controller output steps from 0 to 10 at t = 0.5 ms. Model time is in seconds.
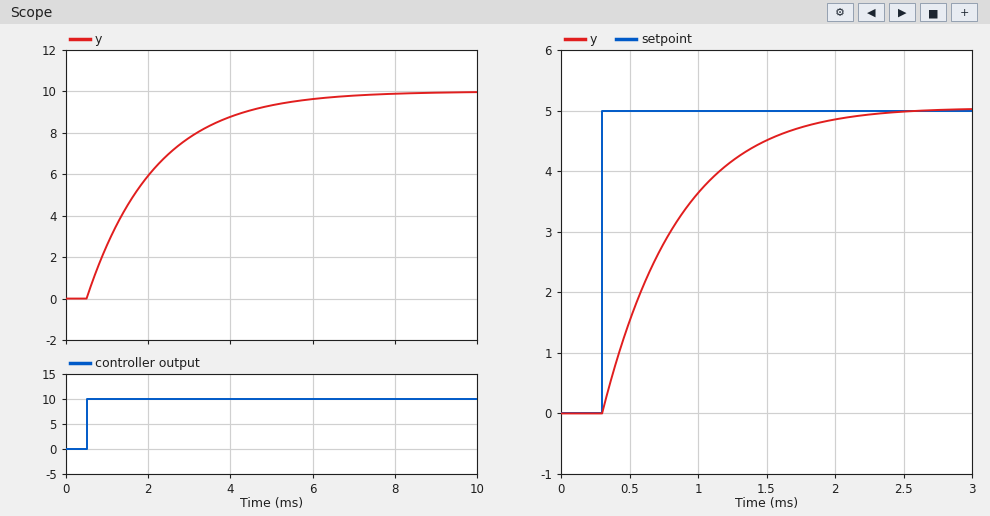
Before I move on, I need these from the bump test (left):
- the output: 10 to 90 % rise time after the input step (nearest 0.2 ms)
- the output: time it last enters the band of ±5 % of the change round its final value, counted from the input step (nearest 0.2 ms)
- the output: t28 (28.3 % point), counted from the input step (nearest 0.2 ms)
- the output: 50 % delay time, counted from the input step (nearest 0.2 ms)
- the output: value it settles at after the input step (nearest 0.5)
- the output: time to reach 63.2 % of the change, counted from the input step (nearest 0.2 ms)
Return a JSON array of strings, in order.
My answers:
["3.6 ms", "5.0 ms", "0.6 ms", "1.2 ms", "10.0", "1.6 ms"]
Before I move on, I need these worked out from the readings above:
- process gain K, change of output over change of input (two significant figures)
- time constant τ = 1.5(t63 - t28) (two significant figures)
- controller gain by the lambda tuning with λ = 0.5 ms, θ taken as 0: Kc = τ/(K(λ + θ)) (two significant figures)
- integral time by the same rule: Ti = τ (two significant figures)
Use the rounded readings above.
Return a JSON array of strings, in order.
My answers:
["1.0", "1.5 ms", "3.0", "1.5 ms"]
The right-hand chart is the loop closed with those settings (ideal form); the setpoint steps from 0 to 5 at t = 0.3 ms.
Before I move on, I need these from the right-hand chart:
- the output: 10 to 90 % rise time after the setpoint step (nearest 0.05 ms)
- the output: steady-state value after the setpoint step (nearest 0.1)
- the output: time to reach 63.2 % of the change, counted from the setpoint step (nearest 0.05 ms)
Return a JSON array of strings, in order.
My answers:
["1.15 ms", "5.0", "0.55 ms"]
